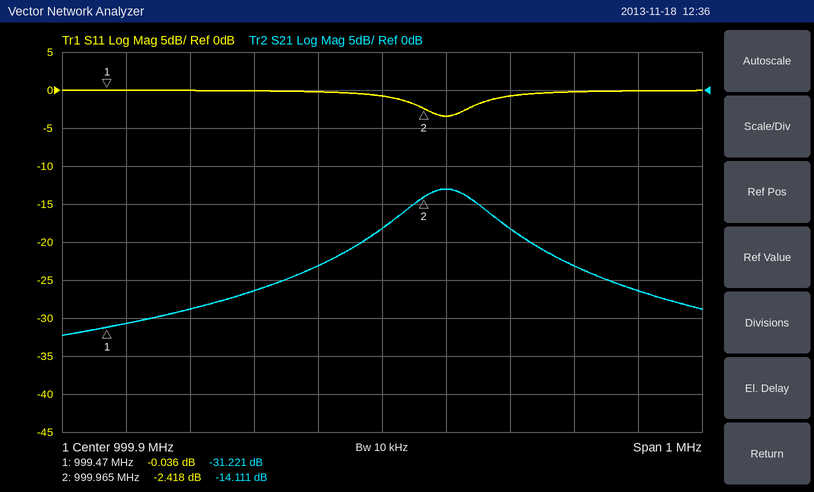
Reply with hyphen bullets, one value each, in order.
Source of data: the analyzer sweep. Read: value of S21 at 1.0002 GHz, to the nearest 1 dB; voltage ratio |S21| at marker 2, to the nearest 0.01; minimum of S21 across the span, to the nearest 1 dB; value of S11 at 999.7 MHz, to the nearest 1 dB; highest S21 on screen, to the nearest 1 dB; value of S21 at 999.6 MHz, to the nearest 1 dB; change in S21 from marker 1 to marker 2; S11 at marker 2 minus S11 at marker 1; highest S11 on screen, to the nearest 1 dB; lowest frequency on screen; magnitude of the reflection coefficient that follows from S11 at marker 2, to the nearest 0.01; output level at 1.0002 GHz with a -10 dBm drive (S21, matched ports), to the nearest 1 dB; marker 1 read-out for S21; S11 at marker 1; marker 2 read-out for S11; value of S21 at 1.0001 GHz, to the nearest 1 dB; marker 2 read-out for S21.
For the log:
- -23 dB
- 0.20
- -32 dB
- 0 dB
- -13 dB
- -29 dB
- 17.110 dB
- -2.382 dB
- 0 dB
- 999.4 MHz
- 0.76
- -33 dBm
- -31.221 dB
- -0.036 dB
- -2.418 dB
- -18 dB
- -14.111 dB
